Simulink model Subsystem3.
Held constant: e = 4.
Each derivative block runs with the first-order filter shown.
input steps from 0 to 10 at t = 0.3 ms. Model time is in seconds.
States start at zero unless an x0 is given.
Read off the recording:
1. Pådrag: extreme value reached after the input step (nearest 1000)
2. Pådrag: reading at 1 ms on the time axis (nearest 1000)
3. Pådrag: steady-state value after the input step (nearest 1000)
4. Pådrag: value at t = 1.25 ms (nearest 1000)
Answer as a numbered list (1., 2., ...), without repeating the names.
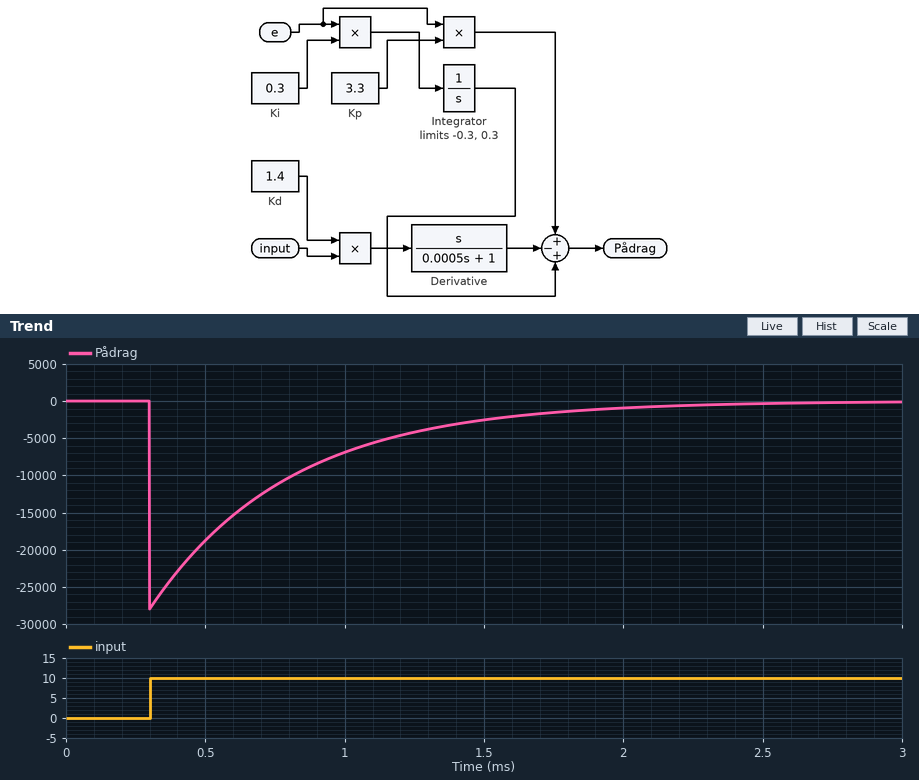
1. -28000
2. -7000
3. 0
4. -4000
